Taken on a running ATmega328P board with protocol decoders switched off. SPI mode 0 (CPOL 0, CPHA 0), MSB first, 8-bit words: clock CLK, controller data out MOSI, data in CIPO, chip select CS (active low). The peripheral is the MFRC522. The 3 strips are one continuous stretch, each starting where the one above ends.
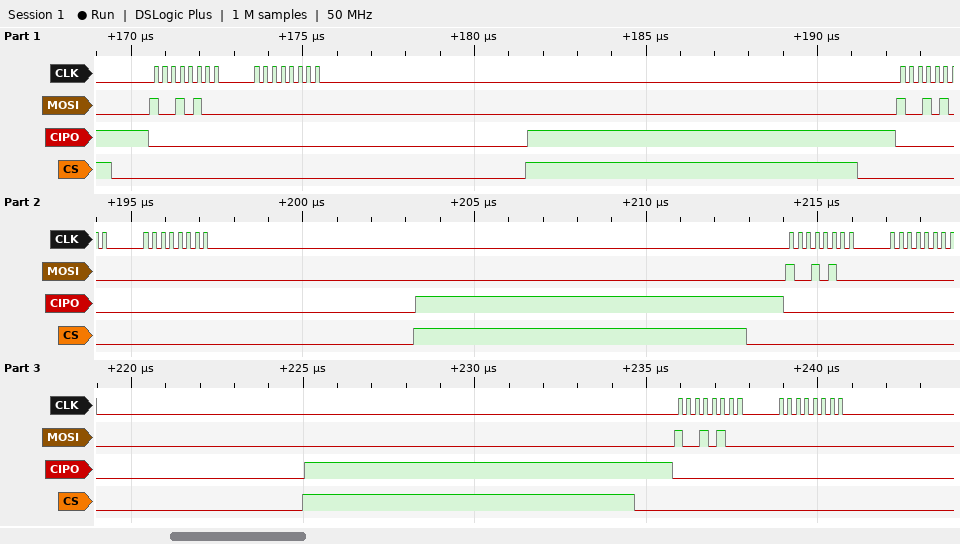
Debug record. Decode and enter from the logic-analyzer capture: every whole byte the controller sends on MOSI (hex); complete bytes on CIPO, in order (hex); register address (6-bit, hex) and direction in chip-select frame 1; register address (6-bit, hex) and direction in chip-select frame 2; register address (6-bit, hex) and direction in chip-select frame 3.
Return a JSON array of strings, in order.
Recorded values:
["94 00 94 00 94 00 94 00", "00 00 00 00 00 00 00 00", "0x0A read", "0x0A read", "0x0A read"]
